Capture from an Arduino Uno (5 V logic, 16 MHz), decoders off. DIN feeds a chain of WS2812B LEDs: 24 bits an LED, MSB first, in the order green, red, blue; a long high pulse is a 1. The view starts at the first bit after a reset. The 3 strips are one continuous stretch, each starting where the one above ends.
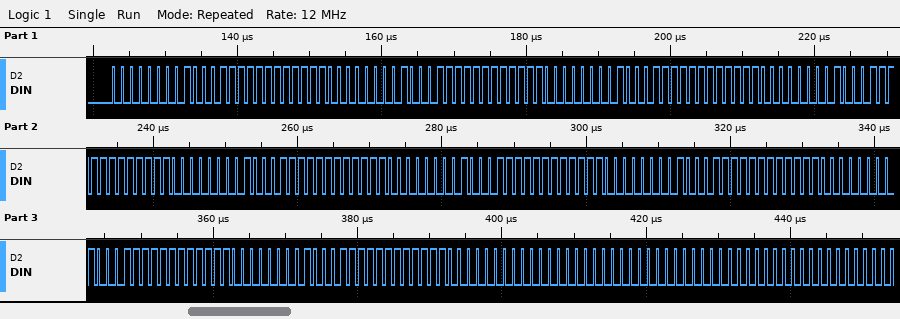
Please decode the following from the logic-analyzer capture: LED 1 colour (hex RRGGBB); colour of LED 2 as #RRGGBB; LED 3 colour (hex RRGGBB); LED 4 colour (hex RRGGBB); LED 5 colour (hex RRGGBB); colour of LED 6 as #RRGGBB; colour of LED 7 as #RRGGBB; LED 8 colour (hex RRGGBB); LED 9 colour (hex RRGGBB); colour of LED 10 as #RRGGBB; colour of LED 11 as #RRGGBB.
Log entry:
#8F00FF
#8F00FF
#8F00FF
#8F00FF
#8F00FF
#8F00FF
#8F00FF
#8F00FF
#8F00FF
#000000
#000000
